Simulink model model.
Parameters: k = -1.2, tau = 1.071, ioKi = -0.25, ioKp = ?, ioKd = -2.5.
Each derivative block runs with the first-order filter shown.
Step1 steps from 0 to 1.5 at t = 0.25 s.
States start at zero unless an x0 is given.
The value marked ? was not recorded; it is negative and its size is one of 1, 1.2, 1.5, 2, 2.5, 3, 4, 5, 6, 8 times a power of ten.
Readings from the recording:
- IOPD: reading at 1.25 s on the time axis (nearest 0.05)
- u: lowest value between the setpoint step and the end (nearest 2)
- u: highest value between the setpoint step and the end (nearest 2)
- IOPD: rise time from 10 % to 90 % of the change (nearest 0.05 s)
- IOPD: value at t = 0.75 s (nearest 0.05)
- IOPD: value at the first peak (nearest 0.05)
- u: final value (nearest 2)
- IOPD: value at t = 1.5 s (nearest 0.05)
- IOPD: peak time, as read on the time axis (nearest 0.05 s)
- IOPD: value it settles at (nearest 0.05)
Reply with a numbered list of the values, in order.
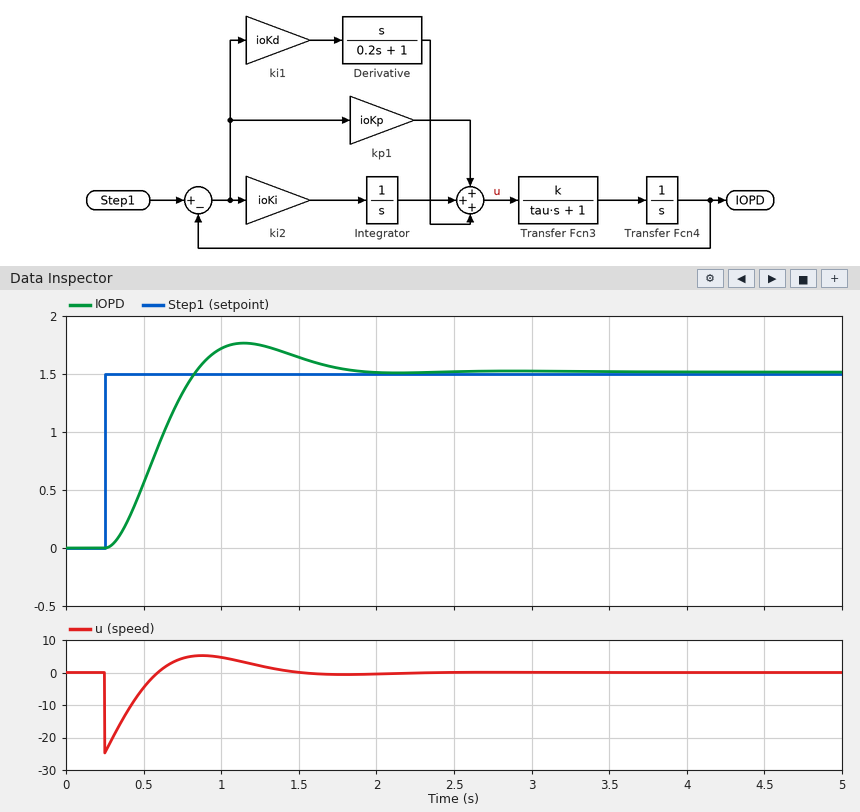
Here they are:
1. 1.75
2. -24
3. 6
4. 0.40 s
5. 1.35
6. 1.75
7. 0
8. 1.65
9. 1.15 s
10. 1.50
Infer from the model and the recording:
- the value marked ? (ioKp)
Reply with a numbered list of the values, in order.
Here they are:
1. -4
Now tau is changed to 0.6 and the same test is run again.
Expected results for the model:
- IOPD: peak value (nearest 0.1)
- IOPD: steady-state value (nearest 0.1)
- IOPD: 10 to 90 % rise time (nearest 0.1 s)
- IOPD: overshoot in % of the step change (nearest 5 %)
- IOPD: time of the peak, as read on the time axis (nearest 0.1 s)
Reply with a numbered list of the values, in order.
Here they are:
1. 1.7
2. 1.5
3. 0.3 s
4. 15 %
5. 0.9 s
